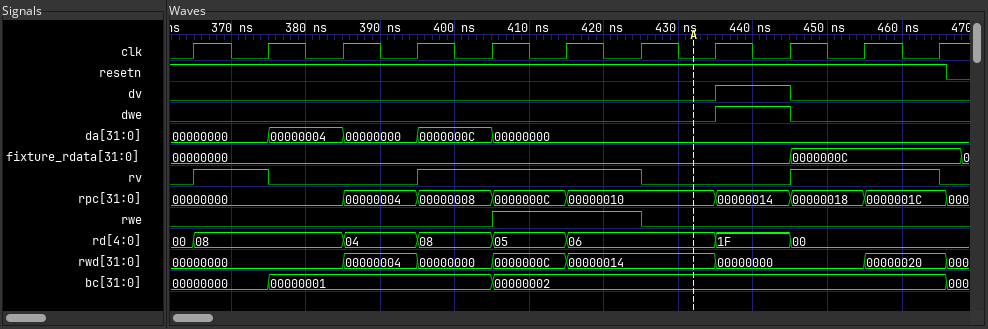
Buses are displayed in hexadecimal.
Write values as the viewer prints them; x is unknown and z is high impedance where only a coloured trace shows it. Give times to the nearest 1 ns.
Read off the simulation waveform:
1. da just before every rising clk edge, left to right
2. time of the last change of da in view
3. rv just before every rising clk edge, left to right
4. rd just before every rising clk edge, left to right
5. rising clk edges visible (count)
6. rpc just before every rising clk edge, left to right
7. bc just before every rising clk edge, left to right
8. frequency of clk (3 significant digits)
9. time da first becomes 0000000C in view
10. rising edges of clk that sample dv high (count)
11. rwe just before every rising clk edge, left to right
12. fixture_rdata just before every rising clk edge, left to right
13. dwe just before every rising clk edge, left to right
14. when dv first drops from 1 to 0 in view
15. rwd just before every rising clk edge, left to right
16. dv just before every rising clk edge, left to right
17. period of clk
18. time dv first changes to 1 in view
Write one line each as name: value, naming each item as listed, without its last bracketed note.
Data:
da just before every rising clk edge, left to right: 00000000, 00000000, 00000004, 00000000, 0000000C, 00000000, 00000000, 00000000, 00000000, 00000000, 00000000
time of the last change of da in view: 405 ns
rv just before every rising clk edge, left to right: 0 1 0 0 1 1 1 0 0 1 1
rd just before every rising clk edge, left to right: 00, 08, 08, 04, 08, 05, 06, 06, 1F, 00, 00
rising clk edges visible: 11
rpc just before every rising clk edge, left to right: 00000000, 00000000, 00000000, 00000004, 00000008, 0000000C, 00000010, 00000010, 00000014, 00000018, 0000001C
bc just before every rising clk edge, left to right: 00000000, 00000000, 00000001, 00000001, 00000001, 00000002, 00000002, 00000002, 00000002, 00000002, 00000002
frequency of clk: 100 MHz
time da first becomes 0000000C in view: 395 ns
rising edges of clk that sample dv high: 1
rwe just before every rising clk edge, left to right: 0 0 0 0 0 1 1 0 0 0 0
fixture_rdata just before every rising clk edge, left to right: 00000000, 00000000, 00000000, 00000000, 00000000, 00000000, 00000000, 00000000, 00000000, 0000000C, 0000000C
dwe just before every rising clk edge, left to right: 0 0 0 0 0 0 0 0 1 0 0
when dv first drops from 1 to 0 in view: 445 ns
rwd just before every rising clk edge, left to right: 00000000, 00000000, 00000000, 00000004, 00000000, 0000000C, 00000014, 00000014, 00000000, 00000000, 00000020
dv just before every rising clk edge, left to right: 0 0 0 0 0 0 0 0 1 0 0
period of clk: 10 ns
time dv first changes to 1 in view: 435 ns
